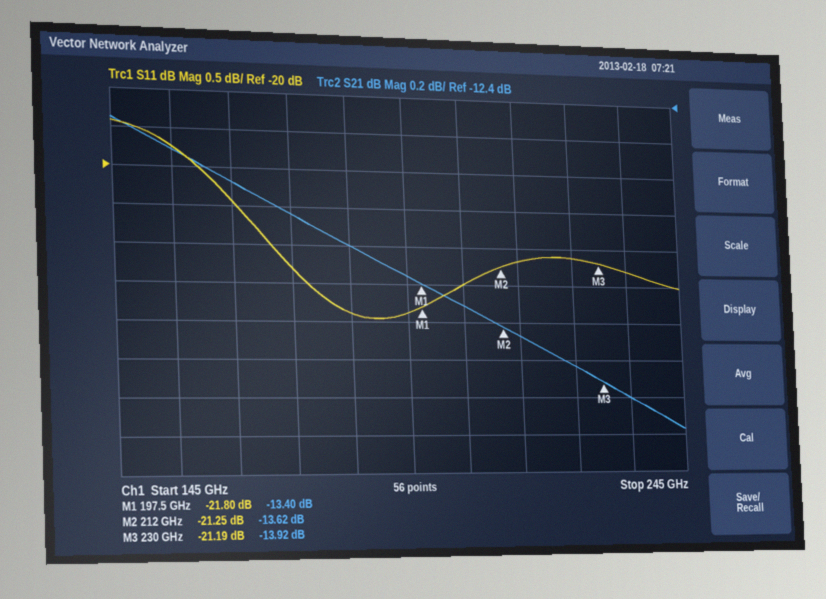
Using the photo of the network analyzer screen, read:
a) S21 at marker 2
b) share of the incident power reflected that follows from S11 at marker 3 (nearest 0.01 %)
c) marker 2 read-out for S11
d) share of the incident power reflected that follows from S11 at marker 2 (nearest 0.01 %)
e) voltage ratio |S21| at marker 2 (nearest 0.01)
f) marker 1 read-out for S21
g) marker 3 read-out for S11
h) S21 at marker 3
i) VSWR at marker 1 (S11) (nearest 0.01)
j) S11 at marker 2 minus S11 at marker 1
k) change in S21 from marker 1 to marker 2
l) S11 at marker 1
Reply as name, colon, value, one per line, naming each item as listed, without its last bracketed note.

S21 at marker 2: -13.62 dB
share of the incident power reflected that follows from S11 at marker 3: 0.76 %
marker 2 read-out for S11: -21.25 dB
share of the incident power reflected that follows from S11 at marker 2: 0.75 %
voltage ratio |S21| at marker 2: 0.21
marker 1 read-out for S21: -13.40 dB
marker 3 read-out for S11: -21.19 dB
S21 at marker 3: -13.92 dB
VSWR at marker 1 (S11): 1.18
S11 at marker 2 minus S11 at marker 1: 0.55 dB
change in S21 from marker 1 to marker 2: -0.22 dB
S11 at marker 1: -21.80 dB
